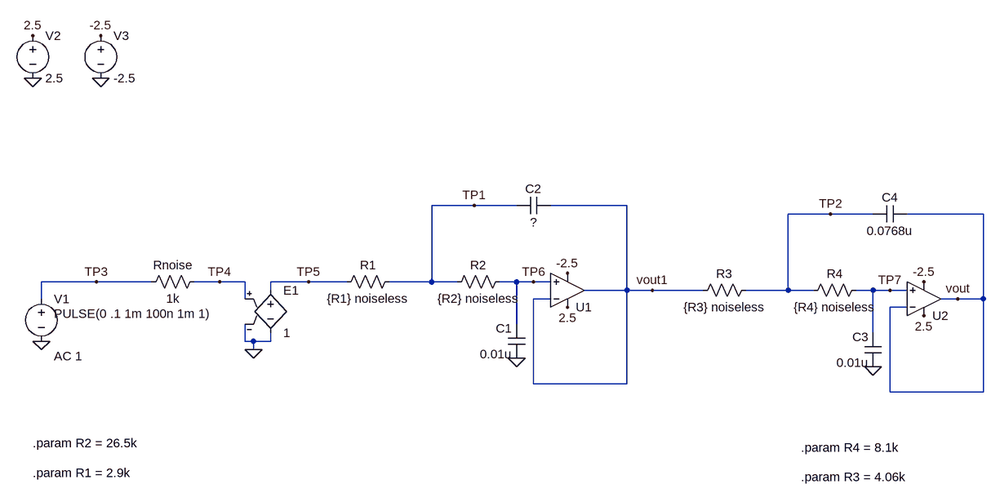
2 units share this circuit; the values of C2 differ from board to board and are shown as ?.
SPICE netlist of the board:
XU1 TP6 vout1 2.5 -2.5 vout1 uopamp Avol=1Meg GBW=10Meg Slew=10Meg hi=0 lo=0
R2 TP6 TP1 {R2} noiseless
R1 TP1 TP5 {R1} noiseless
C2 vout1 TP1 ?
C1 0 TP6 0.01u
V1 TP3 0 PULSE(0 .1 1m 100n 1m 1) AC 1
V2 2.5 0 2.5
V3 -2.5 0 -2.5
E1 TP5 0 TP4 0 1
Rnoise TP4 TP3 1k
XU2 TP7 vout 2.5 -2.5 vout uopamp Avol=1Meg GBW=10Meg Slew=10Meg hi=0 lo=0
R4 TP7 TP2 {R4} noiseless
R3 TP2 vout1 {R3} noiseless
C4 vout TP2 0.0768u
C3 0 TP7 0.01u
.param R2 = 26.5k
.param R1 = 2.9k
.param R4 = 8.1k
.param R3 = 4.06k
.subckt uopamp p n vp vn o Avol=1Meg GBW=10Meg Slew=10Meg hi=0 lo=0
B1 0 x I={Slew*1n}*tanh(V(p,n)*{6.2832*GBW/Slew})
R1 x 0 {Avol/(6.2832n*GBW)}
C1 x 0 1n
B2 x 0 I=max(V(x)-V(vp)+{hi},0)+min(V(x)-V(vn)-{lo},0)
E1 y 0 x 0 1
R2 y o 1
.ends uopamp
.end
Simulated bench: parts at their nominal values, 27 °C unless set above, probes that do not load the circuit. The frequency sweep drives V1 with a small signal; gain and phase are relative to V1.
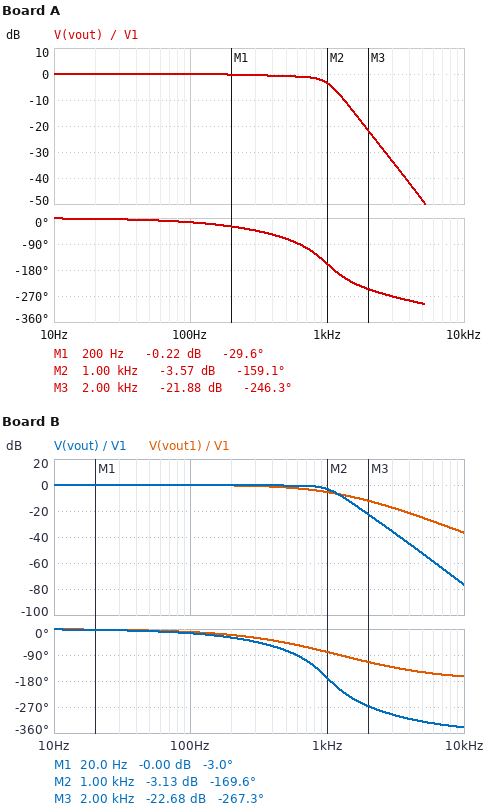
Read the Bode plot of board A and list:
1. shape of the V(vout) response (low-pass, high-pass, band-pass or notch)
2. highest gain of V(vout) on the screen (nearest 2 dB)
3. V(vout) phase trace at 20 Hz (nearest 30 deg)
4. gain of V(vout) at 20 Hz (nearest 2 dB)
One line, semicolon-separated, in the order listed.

low-pass; 0 dB; 0 deg; 0 dB
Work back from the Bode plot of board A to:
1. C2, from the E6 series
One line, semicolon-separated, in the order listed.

10 nF
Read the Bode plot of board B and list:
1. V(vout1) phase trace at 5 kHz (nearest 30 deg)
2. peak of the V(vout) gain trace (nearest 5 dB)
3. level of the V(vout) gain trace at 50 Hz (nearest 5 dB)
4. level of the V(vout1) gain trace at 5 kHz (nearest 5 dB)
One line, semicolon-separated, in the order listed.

-150 deg; 0 dB; 0 dB; -25 dB
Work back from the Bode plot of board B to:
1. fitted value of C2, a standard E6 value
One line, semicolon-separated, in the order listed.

22 nF
